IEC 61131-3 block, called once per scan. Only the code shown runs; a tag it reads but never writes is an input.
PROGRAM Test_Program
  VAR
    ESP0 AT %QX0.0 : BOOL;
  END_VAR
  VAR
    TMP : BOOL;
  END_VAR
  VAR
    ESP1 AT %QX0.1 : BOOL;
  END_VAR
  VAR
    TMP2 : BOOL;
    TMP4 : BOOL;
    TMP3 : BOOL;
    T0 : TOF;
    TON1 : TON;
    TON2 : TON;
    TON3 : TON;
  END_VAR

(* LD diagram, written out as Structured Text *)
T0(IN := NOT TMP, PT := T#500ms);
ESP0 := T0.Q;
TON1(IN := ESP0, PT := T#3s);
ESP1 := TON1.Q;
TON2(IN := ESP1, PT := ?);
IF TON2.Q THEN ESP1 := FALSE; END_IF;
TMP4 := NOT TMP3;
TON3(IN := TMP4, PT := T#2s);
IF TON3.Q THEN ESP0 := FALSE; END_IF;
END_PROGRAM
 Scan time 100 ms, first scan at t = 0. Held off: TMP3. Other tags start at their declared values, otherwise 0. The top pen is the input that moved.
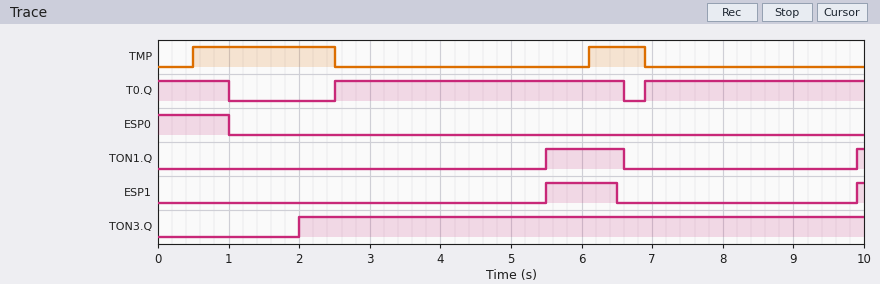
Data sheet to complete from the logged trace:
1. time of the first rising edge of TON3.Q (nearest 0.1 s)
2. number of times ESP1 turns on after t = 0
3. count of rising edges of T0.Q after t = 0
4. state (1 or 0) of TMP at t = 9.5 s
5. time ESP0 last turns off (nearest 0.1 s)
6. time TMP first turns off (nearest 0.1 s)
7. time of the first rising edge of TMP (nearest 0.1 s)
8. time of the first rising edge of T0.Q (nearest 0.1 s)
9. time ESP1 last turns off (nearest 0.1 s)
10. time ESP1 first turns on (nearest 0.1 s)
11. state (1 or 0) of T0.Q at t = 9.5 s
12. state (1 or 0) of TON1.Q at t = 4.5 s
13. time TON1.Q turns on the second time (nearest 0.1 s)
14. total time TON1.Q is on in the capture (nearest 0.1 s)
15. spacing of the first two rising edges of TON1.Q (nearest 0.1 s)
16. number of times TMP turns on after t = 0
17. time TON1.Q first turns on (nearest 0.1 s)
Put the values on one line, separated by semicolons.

2.0 s; 2; 2; 0; 1.0 s; 2.5 s; 0.5 s; 2.5 s; 6.5 s; 5.5 s; 1; 0; 9.9 s; 1.2 s; 4.4 s; 2; 5.5 s
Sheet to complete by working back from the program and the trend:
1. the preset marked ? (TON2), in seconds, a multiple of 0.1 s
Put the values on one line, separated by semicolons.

1.0 s
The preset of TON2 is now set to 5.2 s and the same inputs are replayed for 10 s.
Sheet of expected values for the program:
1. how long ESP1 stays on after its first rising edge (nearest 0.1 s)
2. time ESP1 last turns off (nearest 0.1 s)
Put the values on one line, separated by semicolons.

1.1 s; 6.6 s
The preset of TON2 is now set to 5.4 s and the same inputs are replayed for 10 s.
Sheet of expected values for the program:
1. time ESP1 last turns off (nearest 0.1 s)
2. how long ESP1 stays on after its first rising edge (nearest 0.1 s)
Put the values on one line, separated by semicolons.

6.6 s; 1.1 s
